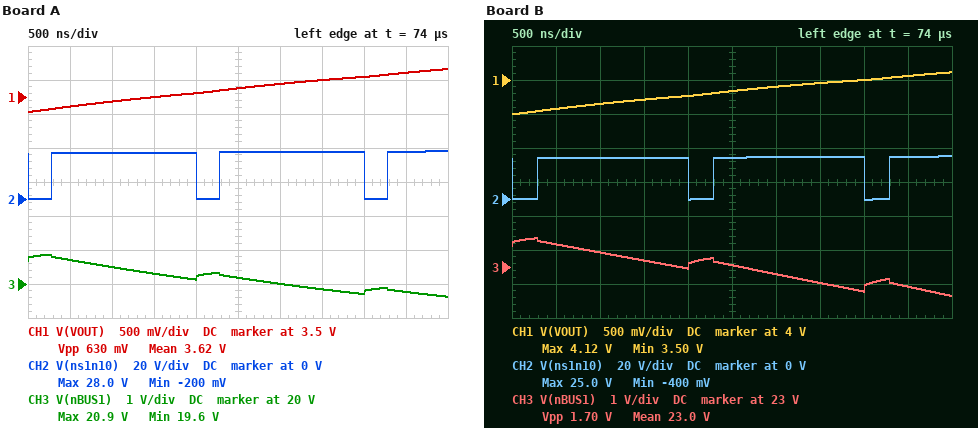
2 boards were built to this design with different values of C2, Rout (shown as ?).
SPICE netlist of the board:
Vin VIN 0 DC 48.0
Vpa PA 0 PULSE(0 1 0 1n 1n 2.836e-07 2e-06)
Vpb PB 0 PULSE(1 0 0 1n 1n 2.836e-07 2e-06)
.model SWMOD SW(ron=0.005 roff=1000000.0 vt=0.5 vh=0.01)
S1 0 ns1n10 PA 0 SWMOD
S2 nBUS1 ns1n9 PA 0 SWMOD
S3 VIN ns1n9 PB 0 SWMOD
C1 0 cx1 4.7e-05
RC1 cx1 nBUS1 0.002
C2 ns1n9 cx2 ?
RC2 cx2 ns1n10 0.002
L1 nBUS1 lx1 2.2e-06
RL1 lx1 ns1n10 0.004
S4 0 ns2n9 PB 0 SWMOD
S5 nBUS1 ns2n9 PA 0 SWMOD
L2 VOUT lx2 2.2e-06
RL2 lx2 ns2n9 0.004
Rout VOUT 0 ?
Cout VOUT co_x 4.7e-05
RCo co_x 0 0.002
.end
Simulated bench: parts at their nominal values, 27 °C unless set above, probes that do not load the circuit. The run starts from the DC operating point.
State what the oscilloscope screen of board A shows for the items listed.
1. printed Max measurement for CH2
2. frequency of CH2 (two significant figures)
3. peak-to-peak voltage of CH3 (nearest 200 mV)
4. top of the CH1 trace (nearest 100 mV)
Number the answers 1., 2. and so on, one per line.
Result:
1. 28.0 V
2. 500 kHz
3. 1.2 V
4. 3.9 V
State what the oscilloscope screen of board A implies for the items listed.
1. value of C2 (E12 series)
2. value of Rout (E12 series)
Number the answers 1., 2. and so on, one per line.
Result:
1. 82 µF
2. 1.8 Ω
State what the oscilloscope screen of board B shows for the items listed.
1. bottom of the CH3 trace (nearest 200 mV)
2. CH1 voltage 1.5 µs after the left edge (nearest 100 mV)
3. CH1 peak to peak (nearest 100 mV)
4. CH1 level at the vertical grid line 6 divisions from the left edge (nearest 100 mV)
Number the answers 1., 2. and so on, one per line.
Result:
1. 22.2 V
2. 3.7 V
3. 600 mV
4. 3.9 V
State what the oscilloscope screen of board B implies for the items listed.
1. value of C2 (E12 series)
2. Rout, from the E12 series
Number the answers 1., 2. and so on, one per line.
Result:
1. 120 µF
2. 0.82 Ω
